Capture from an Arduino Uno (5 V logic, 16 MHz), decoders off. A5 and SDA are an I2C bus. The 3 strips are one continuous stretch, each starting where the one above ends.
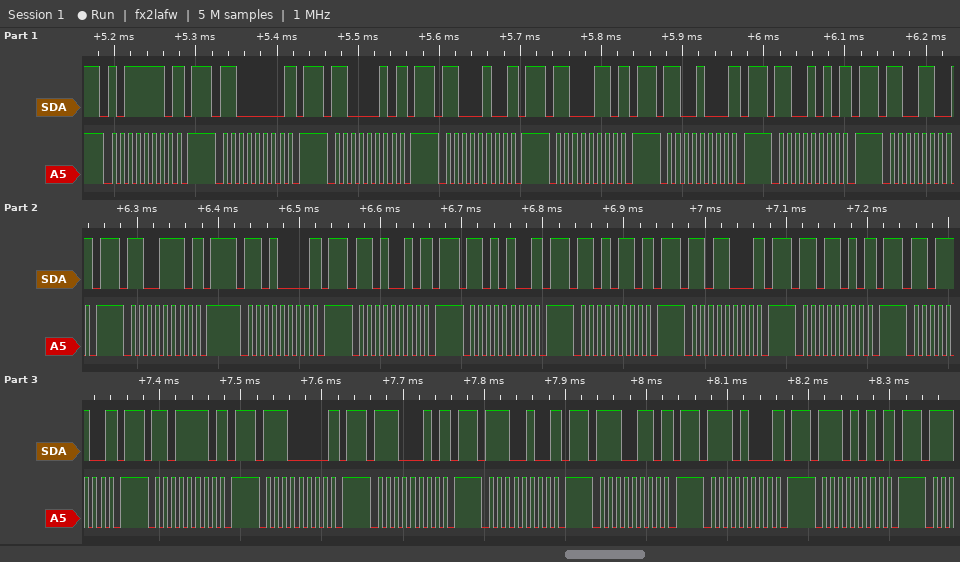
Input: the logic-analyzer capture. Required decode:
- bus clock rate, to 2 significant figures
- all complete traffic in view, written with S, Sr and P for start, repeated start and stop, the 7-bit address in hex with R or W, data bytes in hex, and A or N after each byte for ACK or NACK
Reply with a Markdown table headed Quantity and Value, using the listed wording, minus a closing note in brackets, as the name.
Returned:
| Quantity | Value |
|---|---|
| bus clock rate, to 2 significant figures | 100 kHz |
| all complete traffic in view, written with S, Sr and P for start, repeated start and stop, the 7-bit address in hex with R or W, data bytes in hex, and A or N after each byte for ACK or NACK | S 5FW N P S 60W N P S 61W N P S 62W N P S 63W N P S 64W N P S 65W N P S 66W N P S 67W N P S 68W N P S 69W N P S 6AW N P S 6BW N P S 6CW N P S 6DW N P S 6EW N P S 6FW N P S 70W N P S 71W N P S 72W N P S 73W N P S 74W N P S 75W N P |
